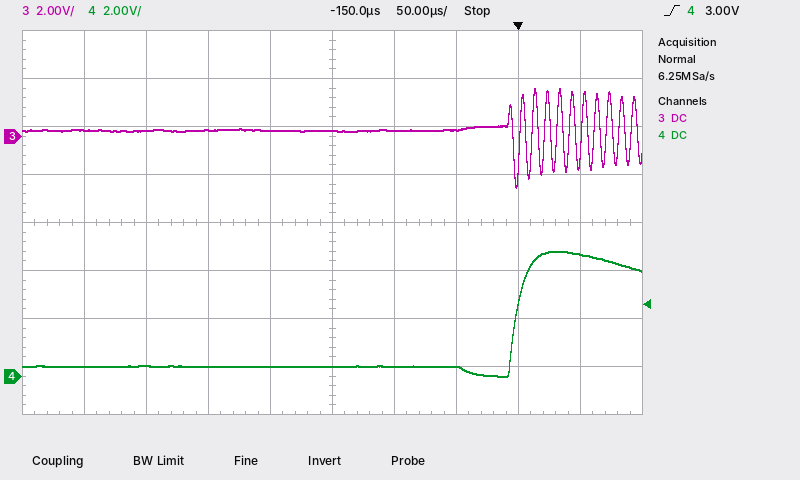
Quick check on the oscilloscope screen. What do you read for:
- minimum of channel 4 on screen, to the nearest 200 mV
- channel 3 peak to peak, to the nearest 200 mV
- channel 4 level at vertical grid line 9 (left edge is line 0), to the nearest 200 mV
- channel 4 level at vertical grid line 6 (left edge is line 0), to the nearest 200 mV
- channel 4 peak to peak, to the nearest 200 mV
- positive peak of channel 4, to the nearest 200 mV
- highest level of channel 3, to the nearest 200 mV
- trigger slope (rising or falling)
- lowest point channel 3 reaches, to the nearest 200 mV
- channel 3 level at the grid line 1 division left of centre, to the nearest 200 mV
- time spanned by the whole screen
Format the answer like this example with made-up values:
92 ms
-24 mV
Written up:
0.0 V
4.2 V
5.0 V
400 mV
5.2 V
5.2 V
2.0 V
rising
-2.2 V
200 mV
500 µs
